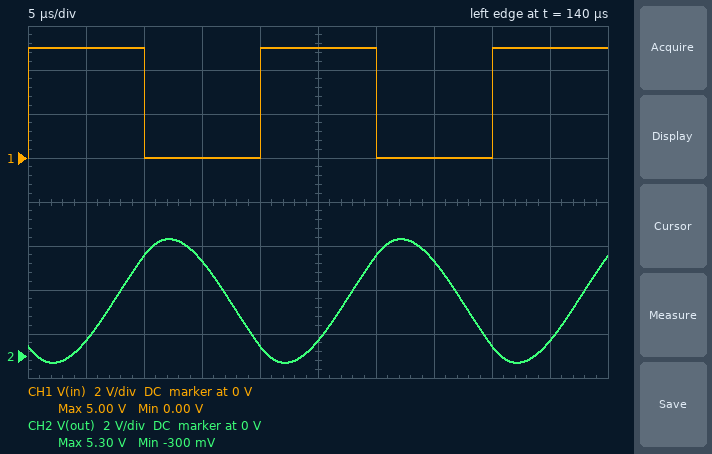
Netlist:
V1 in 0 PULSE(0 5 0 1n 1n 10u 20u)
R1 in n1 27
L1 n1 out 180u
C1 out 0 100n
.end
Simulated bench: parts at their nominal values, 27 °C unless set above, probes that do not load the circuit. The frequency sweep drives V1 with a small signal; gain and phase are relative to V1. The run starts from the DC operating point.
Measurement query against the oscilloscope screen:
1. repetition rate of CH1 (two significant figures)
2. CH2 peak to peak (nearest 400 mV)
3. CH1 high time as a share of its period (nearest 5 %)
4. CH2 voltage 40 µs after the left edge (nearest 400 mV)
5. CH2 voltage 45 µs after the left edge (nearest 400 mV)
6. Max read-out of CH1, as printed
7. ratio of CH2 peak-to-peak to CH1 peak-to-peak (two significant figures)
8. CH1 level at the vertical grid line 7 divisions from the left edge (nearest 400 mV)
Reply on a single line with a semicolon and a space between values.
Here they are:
50 kHz; 5.6 V; 50 %; 400 mV; 800 mV; 5.00 V; 1.1; 0 V
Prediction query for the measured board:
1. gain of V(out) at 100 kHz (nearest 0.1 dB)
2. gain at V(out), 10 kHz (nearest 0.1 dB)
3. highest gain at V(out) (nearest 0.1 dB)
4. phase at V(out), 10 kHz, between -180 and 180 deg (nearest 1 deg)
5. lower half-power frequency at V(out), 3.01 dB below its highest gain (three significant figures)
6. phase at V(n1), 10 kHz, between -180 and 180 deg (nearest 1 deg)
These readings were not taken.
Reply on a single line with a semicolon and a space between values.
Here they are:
-16.0 dB; 0.5 dB; 4.4 dB; -10 deg; 16.5 kHz; -10 deg
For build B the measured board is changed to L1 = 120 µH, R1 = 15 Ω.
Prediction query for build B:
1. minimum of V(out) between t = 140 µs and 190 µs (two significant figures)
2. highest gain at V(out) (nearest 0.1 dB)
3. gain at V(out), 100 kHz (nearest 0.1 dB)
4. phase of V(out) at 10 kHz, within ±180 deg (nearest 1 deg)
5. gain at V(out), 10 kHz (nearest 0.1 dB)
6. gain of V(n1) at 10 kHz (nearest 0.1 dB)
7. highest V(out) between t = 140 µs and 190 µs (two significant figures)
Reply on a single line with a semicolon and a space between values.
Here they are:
-3.9 V; 7.5 dB; -11.7 dB; -6 deg; 0.4 dB; 0 dB; 8.9 V
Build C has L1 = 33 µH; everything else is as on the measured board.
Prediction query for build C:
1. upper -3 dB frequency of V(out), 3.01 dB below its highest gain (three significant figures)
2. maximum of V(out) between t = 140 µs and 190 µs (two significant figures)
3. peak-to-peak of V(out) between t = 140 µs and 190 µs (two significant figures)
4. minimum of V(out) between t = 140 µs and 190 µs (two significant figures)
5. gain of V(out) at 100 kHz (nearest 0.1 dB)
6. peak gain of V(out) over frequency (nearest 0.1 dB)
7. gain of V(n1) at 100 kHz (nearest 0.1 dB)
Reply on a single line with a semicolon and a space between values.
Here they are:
83.2 kHz; 5.2 V; 5.3 V; -160 mV; -4.7 dB; 0 dB; -15.1 dB
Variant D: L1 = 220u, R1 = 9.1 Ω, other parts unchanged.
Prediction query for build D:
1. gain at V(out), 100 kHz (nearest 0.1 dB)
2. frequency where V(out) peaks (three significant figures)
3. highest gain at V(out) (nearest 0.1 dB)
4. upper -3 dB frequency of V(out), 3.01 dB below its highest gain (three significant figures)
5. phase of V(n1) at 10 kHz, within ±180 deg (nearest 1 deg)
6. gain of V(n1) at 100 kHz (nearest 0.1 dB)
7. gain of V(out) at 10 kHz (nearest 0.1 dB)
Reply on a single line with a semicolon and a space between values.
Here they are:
-17.7 dB; 33.6 kHz; 14.3 dB; 36.8 kHz; -4 deg; 0 dB; 0.8 dB
